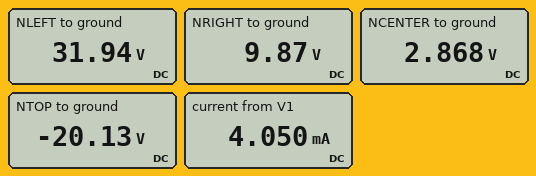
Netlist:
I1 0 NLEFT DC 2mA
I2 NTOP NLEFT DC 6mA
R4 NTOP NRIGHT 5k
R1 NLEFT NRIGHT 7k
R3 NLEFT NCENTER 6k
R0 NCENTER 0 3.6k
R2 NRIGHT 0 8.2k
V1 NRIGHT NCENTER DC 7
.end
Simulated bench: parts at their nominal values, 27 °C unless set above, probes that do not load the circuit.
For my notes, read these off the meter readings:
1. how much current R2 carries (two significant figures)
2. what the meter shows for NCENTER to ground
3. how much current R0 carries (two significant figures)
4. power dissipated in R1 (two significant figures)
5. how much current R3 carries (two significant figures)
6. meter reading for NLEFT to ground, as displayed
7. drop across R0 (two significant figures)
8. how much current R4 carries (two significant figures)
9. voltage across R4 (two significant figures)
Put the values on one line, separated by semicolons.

1.2 mA; 2.868 V; 800 µA; 70 mW; 4.8 mA; 31.94 V; 2.9 V; 6.0 mA; 30 V
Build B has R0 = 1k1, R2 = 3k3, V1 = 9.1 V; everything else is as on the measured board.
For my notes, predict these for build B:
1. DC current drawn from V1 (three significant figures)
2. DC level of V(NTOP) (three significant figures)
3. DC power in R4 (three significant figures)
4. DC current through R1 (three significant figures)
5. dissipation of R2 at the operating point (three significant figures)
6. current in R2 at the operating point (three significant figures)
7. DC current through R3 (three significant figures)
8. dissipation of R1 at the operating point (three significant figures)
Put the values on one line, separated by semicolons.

5.58 mA; -21.5 V; 180 mW; 2.99 mA; 21.8 mW; 2.57 mA; 5.01 mA; 62.7 mW
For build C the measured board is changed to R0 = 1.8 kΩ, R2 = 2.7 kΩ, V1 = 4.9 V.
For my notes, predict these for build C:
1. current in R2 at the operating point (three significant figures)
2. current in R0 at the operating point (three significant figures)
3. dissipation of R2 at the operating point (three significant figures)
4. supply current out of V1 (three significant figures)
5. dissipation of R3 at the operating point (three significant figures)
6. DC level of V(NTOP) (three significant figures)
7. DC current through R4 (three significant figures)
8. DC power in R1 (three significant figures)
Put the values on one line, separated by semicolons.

1.89 mA; 111 µA; 9.63 mW; 4.57 mA; 132 mW; -24.9 V; 6.00 mA; 76.9 mW
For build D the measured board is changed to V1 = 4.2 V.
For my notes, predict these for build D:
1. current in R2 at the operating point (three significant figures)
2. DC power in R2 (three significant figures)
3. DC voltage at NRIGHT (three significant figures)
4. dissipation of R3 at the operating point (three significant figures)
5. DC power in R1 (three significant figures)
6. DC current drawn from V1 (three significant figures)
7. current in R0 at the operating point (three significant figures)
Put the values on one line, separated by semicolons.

966 µA; 7.65 mW; 7.92 V; 129 mW; 79.5 mW; 3.60 mA; 1.03 mA
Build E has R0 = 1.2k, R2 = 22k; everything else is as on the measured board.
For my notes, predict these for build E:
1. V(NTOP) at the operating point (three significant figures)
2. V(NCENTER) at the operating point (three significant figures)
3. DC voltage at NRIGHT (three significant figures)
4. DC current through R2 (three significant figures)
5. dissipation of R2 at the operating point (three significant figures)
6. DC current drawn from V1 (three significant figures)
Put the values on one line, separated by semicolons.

-21.1 V; 1.91 V; 8.91 V; 405 µA; 3.61 mW; 3.25 mA
